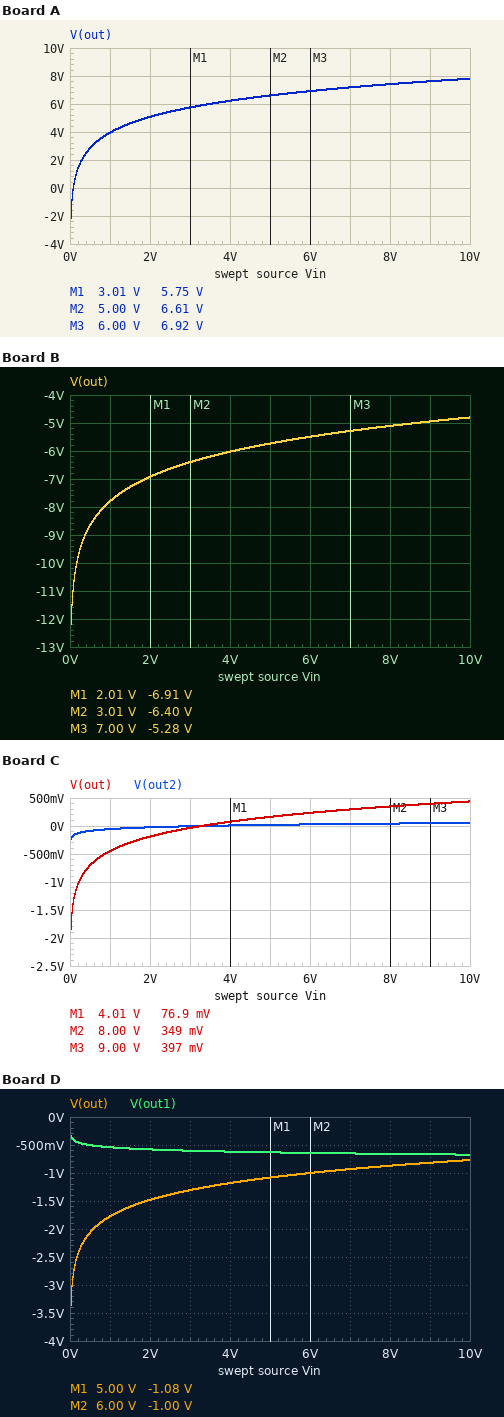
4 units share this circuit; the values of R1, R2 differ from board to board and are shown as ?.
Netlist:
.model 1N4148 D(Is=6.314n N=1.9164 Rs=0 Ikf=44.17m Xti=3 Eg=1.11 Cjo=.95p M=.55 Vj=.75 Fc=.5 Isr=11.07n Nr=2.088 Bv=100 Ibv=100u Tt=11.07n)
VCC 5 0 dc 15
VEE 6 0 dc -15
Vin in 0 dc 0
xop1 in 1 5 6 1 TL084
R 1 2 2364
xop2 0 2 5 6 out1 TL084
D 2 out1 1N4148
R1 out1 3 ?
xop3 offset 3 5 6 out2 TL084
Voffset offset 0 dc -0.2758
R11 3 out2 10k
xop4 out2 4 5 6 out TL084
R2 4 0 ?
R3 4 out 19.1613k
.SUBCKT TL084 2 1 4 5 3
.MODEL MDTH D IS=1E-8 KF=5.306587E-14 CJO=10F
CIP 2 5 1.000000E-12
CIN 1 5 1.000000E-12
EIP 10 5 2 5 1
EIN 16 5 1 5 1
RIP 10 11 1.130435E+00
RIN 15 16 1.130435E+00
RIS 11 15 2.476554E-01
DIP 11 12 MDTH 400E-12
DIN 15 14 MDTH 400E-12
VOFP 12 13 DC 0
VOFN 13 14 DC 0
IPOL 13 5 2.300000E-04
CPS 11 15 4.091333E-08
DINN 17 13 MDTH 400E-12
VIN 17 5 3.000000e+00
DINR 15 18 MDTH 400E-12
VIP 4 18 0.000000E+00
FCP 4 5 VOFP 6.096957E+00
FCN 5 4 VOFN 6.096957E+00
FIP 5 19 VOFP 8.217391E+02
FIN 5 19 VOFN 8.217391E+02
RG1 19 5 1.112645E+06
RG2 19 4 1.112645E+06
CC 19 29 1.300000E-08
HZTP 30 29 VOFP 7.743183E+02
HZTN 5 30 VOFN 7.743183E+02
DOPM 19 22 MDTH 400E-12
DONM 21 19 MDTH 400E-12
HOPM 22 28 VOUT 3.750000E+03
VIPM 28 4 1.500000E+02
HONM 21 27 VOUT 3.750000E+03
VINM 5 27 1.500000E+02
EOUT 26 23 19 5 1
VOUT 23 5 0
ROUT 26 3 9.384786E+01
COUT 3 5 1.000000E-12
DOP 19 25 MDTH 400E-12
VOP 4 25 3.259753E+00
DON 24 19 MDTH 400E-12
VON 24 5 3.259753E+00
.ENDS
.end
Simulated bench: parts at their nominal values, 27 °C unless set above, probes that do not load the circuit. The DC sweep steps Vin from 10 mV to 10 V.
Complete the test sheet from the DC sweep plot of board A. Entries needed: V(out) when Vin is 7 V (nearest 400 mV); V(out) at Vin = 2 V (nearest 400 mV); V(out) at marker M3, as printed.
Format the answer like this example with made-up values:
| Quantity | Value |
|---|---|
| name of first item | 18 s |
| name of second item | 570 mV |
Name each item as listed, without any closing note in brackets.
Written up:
| Quantity | Value |
|---|---|
| V(out) when Vin is 7 V | 7.2 V |
| V(out) at Vin = 2 V | 5.2 V |
| V(out) at marker M3, as printed | 6.92 V |
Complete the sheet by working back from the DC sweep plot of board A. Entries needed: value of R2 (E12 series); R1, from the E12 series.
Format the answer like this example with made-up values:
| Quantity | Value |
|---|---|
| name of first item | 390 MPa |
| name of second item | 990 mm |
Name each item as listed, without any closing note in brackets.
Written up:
| Quantity | Value |
|---|---|
| value of R2 | 1.5 kΩ |
| R1, from the E12 series | 4.7 kΩ |
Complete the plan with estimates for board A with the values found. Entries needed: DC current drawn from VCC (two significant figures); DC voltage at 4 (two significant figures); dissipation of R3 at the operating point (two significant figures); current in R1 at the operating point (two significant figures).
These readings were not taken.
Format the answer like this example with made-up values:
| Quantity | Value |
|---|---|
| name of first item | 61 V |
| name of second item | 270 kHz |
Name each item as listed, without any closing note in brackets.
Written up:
| Quantity | Value |
|---|---|
| DC current drawn from VCC | 5.7 mA |
| DC voltage at 4 | -860 mV |
| dissipation of R3 at the operating point | 6.3 mW |
| current in R1 at the operating point | 59 µA |
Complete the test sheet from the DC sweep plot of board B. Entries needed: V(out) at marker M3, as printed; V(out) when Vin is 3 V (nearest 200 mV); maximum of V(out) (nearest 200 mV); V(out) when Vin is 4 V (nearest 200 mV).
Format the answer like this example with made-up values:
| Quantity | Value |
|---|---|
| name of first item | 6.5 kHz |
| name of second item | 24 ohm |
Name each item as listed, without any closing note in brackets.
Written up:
| Quantity | Value |
|---|---|
| V(out) at marker M3, as printed | -5.28 V |
| V(out) when Vin is 3 V | -6.4 V |
| maximum of V(out) | -4.8 V |
| V(out) when Vin is 4 V | -6.0 V |
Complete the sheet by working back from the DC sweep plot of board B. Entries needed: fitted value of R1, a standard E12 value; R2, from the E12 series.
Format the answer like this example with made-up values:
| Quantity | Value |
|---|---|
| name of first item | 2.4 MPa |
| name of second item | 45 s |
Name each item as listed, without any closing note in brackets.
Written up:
| Quantity | Value |
|---|---|
| fitted value of R1, a standard E12 value | 22 kΩ |
| R2, from the E12 series | 390 Ω |
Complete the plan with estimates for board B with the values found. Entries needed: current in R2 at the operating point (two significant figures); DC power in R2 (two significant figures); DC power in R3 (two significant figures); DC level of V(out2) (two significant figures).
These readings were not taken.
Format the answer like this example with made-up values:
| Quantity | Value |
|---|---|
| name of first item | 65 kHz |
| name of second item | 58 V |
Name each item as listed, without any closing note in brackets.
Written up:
| Quantity | Value |
|---|---|
| current in R2 at the operating point | 650 µA |
| DC power in R2 | 160 µW |
| DC power in R3 | 8.0 mW |
| DC level of V(out2) | -400 mV |
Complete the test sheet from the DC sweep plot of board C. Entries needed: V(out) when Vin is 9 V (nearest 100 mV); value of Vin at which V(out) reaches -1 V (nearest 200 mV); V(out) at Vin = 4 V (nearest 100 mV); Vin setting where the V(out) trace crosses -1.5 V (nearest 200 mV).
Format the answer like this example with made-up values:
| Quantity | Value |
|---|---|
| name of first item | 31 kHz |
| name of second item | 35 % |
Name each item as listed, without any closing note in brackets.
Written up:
| Quantity | Value |
|---|---|
| V(out) when Vin is 9 V | 400 mV |
| value of Vin at which V(out) reaches -1 V | 200 mV |
| V(out) at Vin = 4 V | 100 mV |
| Vin setting where the V(out) trace crosses -1.5 V | 0 V |
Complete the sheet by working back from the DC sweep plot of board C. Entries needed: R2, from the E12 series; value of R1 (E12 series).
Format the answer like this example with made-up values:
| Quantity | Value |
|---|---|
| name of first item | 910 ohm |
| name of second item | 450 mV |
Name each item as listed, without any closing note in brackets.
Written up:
| Quantity | Value |
|---|---|
| R2, from the E12 series | 2.7 kΩ |
| value of R1 | 12 kΩ |
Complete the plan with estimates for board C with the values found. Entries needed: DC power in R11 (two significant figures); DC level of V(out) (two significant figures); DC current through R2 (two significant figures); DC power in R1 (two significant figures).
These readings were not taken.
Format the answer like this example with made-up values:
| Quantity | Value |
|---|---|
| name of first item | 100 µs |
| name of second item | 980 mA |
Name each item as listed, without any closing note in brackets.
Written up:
| Quantity | Value |
|---|---|
| DC power in R11 | 5.3 µW |
| DC level of V(out) | -4.1 V |
| DC current through R2 | 190 µA |
| DC power in R1 | 6.3 µW |
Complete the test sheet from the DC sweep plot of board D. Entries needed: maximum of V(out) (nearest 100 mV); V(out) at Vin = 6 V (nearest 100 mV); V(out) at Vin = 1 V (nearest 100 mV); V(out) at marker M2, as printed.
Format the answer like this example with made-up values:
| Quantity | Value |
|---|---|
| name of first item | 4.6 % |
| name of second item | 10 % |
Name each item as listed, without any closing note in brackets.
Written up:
| Quantity | Value |
|---|---|
| maximum of V(out) | -800 mV |
| V(out) at Vin = 6 V | -1.0 V |
| V(out) at Vin = 1 V | -1.8 V |
| V(out) at marker M2, as printed | -1.00 V |
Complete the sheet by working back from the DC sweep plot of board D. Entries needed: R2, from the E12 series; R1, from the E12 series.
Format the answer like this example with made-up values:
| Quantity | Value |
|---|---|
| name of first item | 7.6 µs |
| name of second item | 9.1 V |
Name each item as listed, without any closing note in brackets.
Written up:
| Quantity | Value |
|---|---|
| R2, from the E12 series | 1.5 kΩ |
| R1, from the E12 series | 18 kΩ |
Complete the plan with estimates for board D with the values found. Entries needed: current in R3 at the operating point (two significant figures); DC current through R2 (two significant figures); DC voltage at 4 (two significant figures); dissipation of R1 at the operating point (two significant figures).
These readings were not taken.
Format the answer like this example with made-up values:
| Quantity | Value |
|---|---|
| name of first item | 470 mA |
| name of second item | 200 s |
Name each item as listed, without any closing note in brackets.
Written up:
| Quantity | Value |
|---|---|
| current in R3 at the operating point | 290 µA |
| DC current through R2 | 290 µA |
| DC voltage at 4 | -430 mV |
| dissipation of R1 at the operating point | 4.2 µW |
